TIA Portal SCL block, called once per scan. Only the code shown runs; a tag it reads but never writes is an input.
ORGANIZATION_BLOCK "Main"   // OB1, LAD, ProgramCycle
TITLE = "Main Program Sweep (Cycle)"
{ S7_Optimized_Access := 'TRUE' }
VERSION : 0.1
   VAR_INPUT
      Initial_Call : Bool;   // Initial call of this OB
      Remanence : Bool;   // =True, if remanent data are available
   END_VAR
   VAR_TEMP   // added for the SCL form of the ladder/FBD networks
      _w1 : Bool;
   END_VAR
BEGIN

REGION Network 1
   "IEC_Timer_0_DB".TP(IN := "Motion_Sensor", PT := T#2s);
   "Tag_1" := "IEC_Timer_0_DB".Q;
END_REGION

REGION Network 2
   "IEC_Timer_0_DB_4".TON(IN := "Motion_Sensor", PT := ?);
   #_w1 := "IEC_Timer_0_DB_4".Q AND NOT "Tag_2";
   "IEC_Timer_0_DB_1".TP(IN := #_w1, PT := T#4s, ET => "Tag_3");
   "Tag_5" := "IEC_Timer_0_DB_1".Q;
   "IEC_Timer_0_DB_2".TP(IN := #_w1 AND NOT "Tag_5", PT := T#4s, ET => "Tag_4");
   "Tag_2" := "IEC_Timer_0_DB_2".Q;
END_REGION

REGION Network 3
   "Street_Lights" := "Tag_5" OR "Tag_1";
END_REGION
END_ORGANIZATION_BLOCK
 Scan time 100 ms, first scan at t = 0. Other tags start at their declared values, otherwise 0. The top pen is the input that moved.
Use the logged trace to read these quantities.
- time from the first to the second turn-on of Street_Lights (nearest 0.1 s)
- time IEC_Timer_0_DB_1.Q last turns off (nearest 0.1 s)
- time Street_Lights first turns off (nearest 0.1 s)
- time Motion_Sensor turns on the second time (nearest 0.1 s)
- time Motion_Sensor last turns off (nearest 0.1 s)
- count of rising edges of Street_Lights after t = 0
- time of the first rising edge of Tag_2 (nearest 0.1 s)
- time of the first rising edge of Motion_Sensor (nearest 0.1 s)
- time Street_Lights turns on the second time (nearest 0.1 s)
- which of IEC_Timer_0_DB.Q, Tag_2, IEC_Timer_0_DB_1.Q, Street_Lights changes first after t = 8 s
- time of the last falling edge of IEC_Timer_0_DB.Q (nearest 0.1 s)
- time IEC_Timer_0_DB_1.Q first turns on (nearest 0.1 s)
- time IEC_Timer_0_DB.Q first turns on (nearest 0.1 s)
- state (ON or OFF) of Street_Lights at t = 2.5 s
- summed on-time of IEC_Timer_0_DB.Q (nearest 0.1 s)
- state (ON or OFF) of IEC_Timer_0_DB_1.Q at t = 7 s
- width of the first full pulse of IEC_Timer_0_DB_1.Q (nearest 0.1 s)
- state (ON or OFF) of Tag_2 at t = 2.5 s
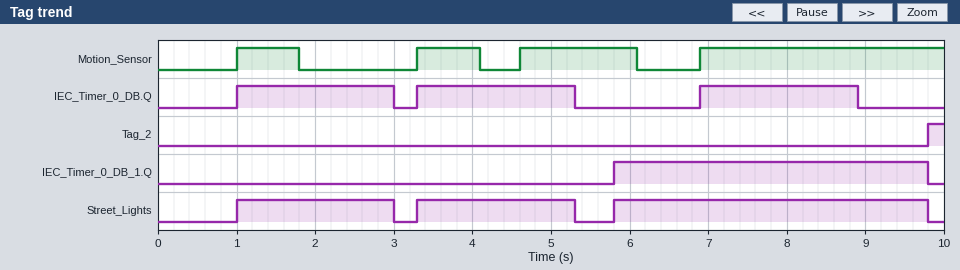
2.3 s
9.8 s
3.0 s
3.3 s
6.1 s
3
9.8 s
1.0 s
3.3 s
IEC_Timer_0_DB.Q
8.9 s
5.8 s
1.0 s
ON
6.0 s
ON
4.0 s
OFF
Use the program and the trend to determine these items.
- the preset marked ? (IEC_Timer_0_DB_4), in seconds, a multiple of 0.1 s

1.2 s
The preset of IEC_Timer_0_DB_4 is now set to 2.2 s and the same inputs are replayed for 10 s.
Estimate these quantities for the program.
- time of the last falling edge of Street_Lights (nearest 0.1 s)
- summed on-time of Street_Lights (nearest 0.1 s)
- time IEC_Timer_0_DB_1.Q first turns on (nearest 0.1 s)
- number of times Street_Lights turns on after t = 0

8.9 s
6.9 s
9.1 s
4
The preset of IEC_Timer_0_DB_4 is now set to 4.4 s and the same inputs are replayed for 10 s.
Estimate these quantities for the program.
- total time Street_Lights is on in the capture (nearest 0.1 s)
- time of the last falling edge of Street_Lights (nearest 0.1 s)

6.0 s
8.9 s
